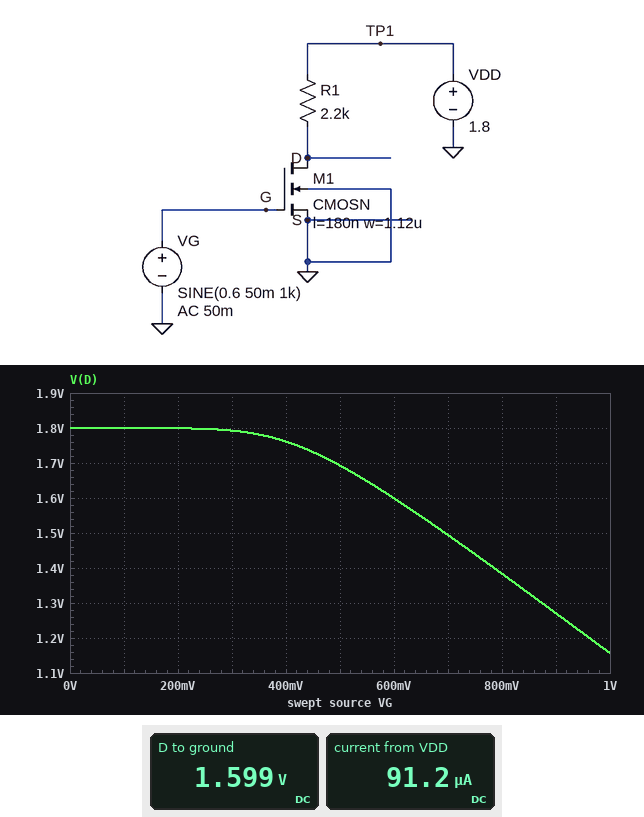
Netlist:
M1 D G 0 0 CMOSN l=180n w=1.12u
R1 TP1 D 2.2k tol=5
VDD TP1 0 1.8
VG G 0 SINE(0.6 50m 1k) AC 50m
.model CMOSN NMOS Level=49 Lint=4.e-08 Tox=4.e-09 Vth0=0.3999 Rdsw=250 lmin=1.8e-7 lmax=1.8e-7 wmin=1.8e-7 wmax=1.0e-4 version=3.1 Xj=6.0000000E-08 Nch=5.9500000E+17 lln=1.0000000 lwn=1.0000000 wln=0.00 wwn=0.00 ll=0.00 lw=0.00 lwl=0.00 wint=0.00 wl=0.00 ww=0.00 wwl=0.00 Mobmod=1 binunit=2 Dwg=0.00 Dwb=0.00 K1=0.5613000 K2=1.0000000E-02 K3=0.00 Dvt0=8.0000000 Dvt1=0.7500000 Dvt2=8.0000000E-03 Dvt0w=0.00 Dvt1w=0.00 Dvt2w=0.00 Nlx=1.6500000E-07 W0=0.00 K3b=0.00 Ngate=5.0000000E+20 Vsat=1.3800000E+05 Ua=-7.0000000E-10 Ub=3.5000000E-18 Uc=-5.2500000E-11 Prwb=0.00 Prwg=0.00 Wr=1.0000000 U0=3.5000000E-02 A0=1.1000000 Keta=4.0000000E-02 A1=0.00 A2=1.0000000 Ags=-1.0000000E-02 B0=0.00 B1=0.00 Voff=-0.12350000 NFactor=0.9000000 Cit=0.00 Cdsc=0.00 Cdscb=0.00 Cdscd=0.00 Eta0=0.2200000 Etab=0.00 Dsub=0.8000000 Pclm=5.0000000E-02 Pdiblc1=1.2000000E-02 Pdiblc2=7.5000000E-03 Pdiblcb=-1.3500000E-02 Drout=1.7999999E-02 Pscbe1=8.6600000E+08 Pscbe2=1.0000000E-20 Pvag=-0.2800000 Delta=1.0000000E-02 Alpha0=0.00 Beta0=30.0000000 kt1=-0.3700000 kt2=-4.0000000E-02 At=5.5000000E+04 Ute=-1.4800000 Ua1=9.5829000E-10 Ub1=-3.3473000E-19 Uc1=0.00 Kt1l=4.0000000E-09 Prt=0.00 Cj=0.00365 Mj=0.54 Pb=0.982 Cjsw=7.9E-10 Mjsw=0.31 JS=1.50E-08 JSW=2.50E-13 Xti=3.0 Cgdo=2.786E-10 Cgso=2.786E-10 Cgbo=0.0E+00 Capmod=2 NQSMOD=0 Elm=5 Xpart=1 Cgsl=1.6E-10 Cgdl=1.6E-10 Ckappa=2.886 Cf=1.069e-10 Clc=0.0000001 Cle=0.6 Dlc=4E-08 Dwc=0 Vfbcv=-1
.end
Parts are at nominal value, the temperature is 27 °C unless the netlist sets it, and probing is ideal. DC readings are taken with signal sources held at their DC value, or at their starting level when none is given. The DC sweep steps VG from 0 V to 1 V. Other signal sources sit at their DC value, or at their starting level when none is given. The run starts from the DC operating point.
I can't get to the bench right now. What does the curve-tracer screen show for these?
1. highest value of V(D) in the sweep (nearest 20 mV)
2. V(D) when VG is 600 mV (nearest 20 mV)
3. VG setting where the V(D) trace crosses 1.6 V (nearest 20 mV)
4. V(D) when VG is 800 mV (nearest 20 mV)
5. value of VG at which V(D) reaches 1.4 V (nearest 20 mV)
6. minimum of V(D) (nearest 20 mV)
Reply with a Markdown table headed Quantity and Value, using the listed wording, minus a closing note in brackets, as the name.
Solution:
| Quantity | Value |
|---|---|
| highest value of V(D) in the sweep | 1.80 V |
| V(D) when VG is 600 mV | 1.60 V |
| VG setting where the V(D) trace crosses 1.6 V | 600 mV |
| V(D) when VG is 800 mV | 1.38 V |
| value of VG at which V(D) reaches 1.4 V | 780 mV |
| minimum of V(D) | 1.16 V |
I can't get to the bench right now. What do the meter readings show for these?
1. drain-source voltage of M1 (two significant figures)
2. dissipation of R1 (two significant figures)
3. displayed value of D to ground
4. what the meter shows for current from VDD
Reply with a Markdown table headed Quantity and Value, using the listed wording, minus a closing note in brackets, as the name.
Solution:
| Quantity | Value |
|---|---|
| drain-source voltage of M1 | 1.6 V |
| dissipation of R1 | 18 µW |
| displayed value of D to ground | 1.599 V |
| what the meter shows for current from VDD | 91.2 µA |
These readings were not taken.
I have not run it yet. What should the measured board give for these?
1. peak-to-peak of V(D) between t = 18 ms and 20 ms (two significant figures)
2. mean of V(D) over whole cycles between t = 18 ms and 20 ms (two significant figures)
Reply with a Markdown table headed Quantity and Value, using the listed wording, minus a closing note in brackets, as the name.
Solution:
| Quantity | Value |
|---|---|
| peak-to-peak of V(D) between t = 18 ms and 20 ms | 100 mV |
| mean of V(D) over whole cycles between t = 18 ms and 20 ms | 1.6 V |
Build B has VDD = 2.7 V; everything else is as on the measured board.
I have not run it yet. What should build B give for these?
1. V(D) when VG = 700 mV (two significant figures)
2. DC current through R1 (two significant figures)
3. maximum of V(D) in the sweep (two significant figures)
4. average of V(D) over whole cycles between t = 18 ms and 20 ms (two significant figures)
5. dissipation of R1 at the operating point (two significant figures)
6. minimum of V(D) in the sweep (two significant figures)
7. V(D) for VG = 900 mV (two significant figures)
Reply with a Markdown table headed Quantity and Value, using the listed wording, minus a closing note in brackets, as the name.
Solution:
| Quantity | Value |
|---|---|
| V(D) when VG = 700 mV | 2.3 V |
| DC current through R1 | 130 µA |
| maximum of V(D) in the sweep | 2.7 V |
| average of V(D) over whole cycles between t = 18 ms and 20 ms | 2.4 V |
| dissipation of R1 at the operating point | 37 µW |
| minimum of V(D) in the sweep | 1.9 V |
| V(D) for VG = 900 mV | 2.1 V |
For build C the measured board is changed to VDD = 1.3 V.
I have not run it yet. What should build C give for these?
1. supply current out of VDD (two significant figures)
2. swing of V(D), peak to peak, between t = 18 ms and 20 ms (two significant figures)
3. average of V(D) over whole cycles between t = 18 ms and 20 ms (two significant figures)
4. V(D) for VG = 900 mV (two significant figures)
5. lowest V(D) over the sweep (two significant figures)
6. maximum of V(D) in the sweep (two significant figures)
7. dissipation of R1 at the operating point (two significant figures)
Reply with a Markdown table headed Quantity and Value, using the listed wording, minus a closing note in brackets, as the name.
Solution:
| Quantity | Value |
|---|---|
| supply current out of VDD | 72 µA |
| swing of V(D), peak to peak, between t = 18 ms and 20 ms | 91 mV |
| average of V(D) over whole cycles between t = 18 ms and 20 ms | 1.1 V |
| V(D) for VG = 900 mV | 830 mV |
| lowest V(D) over the sweep | 720 mV |
| maximum of V(D) in the sweep | 1.3 V |
| dissipation of R1 at the operating point | 11 µW |
